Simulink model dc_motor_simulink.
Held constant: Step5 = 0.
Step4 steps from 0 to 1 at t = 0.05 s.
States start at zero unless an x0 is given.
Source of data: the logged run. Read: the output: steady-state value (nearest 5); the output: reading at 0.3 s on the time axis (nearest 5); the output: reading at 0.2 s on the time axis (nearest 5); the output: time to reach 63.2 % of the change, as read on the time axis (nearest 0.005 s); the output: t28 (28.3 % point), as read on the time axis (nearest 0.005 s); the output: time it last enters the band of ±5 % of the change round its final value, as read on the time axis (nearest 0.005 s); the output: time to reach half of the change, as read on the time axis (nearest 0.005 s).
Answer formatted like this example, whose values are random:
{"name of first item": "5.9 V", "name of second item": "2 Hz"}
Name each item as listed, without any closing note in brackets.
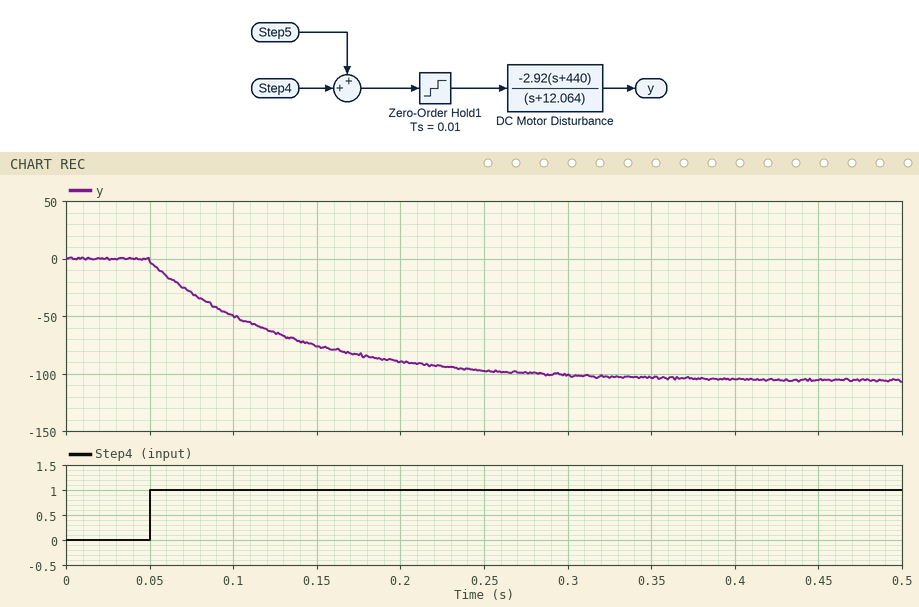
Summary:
{"the output: steady-state value": "-105", "the output: reading at 0.3 s on the time axis": "-100", "the output: reading at 0.2 s on the time axis": "-90", "the output: time to reach 63.2 % of the change, as read on the time axis": "0.130 s", "the output: t28 (28.3 % point), as read on the time axis": "0.075 s", "the output: time it last enters the band of ±5 % of the change round its final value, as read on the time axis": "0.295 s", "the output: time to reach half of the change, as read on the time axis": "0.105 s"}
